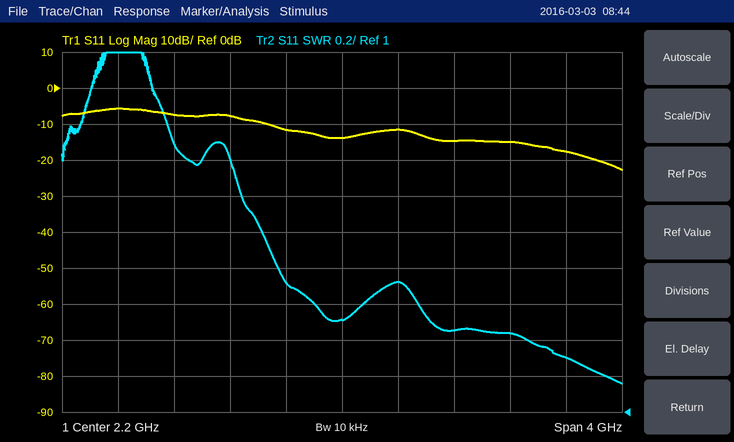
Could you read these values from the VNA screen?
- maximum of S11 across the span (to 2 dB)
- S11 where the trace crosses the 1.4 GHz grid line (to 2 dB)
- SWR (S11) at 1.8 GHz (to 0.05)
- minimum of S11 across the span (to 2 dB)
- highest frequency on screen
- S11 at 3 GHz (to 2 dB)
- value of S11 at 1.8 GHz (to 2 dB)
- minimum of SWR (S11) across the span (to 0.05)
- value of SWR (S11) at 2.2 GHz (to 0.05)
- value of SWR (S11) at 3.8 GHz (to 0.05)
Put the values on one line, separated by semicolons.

-6 dB; -8 dB; 1.70; -22 dB; 4.2 GHz; -14 dB; -12 dB; 1.15; 1.50; 1.30
